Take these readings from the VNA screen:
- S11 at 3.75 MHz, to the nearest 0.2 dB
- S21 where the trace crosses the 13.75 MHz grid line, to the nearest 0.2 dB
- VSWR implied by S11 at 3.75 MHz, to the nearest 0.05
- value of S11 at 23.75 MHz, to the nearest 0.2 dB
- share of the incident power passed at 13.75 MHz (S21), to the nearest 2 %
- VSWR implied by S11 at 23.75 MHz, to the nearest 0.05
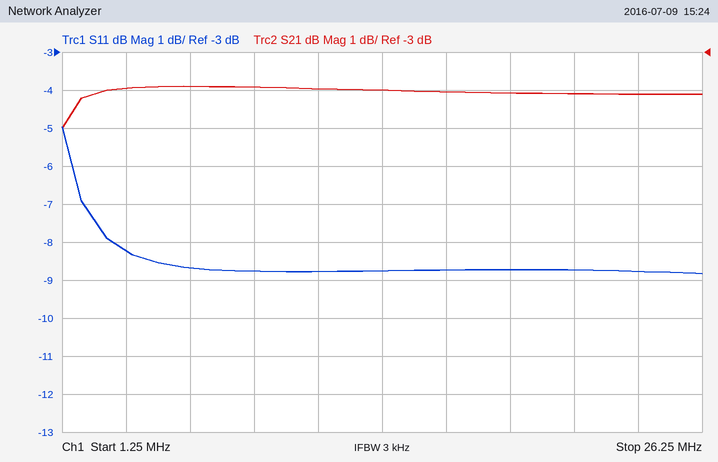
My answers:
-8.2 dB
-4.0 dB
2.25
-8.8 dB
40 %
2.15
